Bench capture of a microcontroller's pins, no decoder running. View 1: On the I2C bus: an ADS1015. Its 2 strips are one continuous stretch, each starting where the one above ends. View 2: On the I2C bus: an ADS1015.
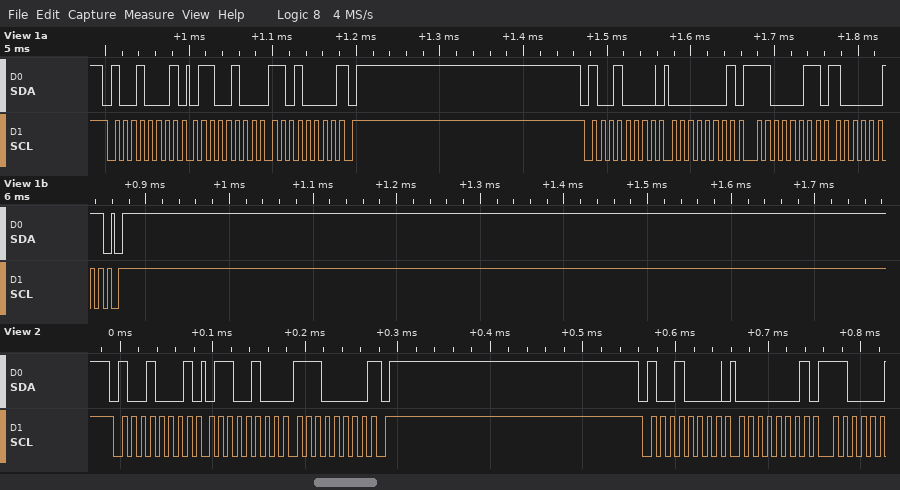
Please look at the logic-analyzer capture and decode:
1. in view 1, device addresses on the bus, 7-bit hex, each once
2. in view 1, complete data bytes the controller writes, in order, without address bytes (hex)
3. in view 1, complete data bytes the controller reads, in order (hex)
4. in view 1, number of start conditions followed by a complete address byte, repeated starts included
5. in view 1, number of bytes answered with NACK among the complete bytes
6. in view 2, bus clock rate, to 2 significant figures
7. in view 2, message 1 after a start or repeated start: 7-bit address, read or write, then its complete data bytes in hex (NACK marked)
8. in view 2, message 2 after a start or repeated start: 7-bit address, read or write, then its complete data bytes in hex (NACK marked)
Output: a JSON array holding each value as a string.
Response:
["0x48", "01 C3 83", "64 D0", "2", "1", "100 kHz", "0x48 read: 64 E0 NACK", "0x48 write: 01"]
